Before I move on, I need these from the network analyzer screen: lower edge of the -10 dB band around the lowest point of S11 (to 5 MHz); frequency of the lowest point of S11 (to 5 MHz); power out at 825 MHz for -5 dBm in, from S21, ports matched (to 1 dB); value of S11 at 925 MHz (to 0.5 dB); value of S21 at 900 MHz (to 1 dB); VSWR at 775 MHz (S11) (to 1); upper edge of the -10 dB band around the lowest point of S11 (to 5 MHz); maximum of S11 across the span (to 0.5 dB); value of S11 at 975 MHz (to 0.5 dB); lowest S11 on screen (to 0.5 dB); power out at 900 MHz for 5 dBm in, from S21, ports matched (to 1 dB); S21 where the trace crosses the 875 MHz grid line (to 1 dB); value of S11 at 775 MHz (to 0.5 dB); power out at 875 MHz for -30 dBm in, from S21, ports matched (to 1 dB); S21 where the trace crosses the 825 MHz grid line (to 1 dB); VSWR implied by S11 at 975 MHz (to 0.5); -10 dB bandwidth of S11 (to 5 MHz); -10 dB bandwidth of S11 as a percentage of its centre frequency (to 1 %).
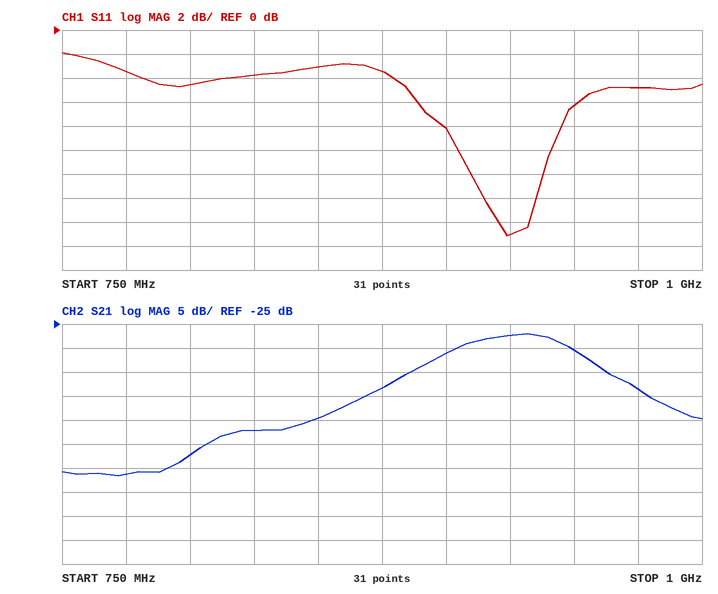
905 MHz
925 MHz
-52 dBm
-17.0 dB
-31 dB
5
940 MHz
-2.0 dB
-5.0 dB
-17.0 dB
-26 dBm
-38 dB
-3.5 dB
-68 dBm
-47 dB
3.5
35 MHz
4 %
